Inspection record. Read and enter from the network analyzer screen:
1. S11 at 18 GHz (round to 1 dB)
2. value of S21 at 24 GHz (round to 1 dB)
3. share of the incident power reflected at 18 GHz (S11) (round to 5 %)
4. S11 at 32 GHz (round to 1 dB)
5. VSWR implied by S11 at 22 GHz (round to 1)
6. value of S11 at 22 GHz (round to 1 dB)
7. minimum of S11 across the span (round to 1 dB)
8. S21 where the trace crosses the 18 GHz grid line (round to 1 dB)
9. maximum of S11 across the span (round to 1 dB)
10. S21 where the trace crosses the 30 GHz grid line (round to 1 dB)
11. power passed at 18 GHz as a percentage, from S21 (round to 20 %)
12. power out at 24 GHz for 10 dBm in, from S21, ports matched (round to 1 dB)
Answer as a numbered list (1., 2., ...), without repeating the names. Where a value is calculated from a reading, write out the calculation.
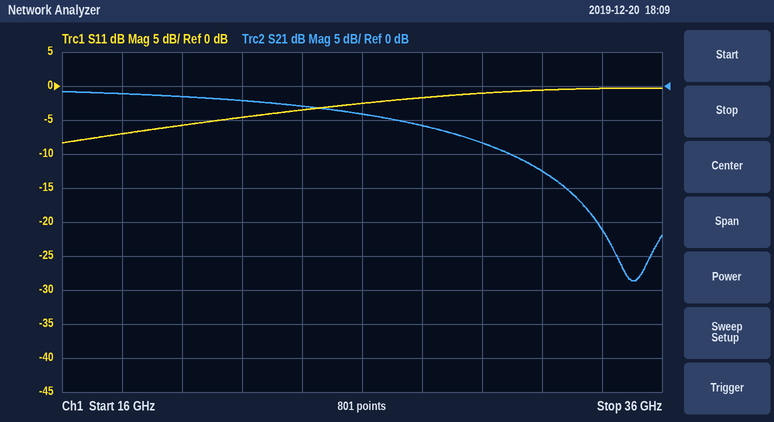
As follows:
1. -7 dB
2. -3 dB
3. 10^(-7/10) ≈ 20 %
4. -1 dB
5. |Γ| = 10^(-5/20) = 0.5623; VSWR = (1 + 0.5623)/(1 − 0.5623) ≈ 4
6. -5 dB
7. -8 dB
8. -1 dB
9. 0 dB
10. -8 dB
11. 10^(-1/10) ≈ 79.4 %, so 80 % to the nearest 20 %
12. 10 dBm + (-3 dB) = 7 dBm
